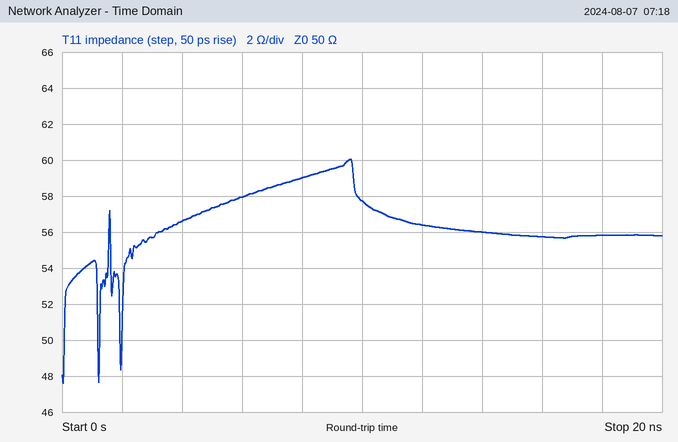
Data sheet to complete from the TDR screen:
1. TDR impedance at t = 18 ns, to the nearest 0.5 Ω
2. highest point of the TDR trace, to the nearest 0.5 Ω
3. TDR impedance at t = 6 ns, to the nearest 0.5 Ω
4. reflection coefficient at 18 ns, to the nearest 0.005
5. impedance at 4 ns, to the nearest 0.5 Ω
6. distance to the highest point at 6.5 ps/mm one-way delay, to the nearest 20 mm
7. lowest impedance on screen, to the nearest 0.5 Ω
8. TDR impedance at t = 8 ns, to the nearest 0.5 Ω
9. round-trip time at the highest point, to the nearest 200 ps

56.0 Ω
60.0 Ω
58.0 Ω
+0.055
56.5 Ω
740 mm
47.5 Ω
59.0 Ω
9.6 ns
